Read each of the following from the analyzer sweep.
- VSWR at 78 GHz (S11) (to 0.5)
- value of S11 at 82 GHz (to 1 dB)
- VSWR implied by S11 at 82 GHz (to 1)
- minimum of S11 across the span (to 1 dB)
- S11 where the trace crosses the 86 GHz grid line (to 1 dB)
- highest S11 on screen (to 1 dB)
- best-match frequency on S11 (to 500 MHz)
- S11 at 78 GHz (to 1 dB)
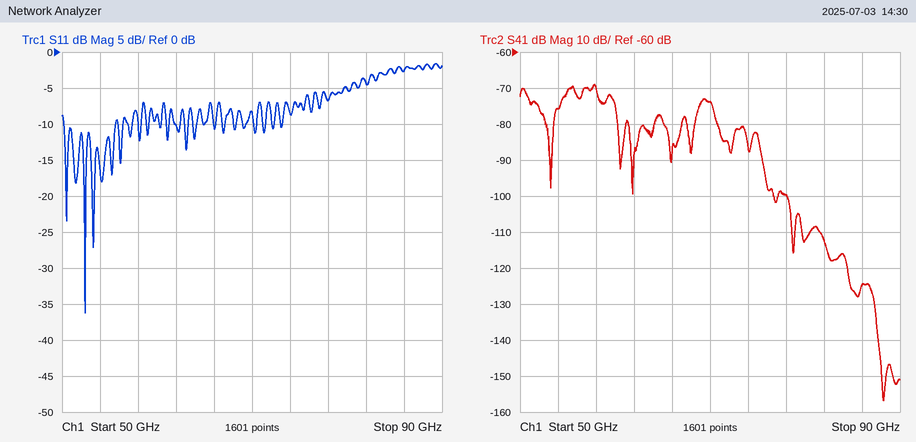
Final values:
2.5
-4 dB
4
-36 dB
-3 dB
-2 dB
52.5 GHz
-7 dB
